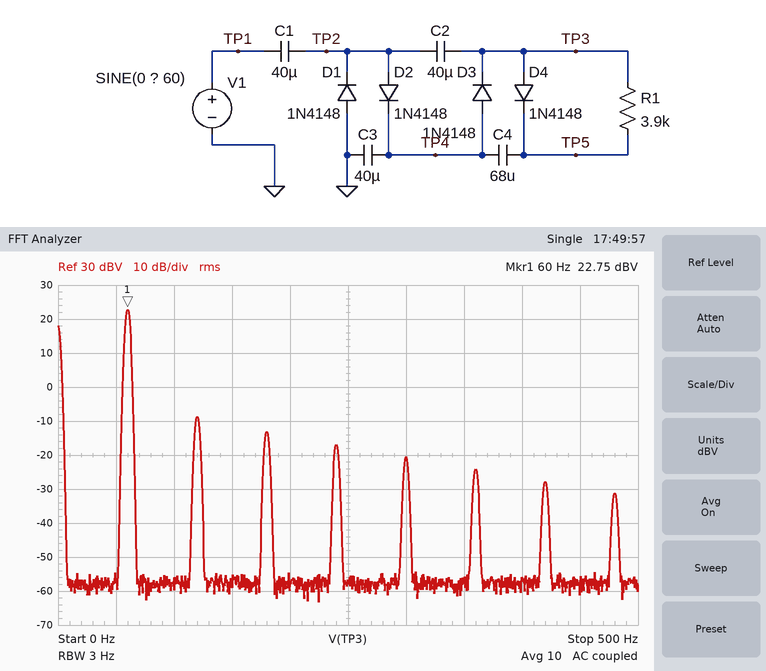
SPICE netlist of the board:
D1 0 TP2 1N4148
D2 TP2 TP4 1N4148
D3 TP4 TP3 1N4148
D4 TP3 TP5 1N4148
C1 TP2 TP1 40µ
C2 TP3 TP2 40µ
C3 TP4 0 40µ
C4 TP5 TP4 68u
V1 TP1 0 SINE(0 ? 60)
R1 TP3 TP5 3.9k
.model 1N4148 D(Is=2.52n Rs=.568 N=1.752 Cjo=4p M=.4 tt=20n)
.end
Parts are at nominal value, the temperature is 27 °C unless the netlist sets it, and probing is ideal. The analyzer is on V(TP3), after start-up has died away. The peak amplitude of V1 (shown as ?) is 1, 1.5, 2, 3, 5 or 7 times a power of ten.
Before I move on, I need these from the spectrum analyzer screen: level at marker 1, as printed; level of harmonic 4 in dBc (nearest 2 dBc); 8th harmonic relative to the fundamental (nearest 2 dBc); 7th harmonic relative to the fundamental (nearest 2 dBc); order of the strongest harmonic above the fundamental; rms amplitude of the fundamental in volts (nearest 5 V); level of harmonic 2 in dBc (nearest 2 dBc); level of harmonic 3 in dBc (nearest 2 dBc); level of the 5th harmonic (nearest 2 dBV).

22.75 dBV
-40 dBc
-54 dBc
-50 dBc
2
15 V
-32 dBc
-36 dBc
-20 dBV
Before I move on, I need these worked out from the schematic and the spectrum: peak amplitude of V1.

20 V
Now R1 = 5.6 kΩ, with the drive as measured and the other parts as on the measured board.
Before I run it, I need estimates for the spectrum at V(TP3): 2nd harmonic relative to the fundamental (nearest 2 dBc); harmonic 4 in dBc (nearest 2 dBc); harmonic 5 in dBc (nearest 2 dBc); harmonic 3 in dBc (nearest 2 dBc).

-34 dBc
-42 dBc
-44 dBc
-38 dBc
